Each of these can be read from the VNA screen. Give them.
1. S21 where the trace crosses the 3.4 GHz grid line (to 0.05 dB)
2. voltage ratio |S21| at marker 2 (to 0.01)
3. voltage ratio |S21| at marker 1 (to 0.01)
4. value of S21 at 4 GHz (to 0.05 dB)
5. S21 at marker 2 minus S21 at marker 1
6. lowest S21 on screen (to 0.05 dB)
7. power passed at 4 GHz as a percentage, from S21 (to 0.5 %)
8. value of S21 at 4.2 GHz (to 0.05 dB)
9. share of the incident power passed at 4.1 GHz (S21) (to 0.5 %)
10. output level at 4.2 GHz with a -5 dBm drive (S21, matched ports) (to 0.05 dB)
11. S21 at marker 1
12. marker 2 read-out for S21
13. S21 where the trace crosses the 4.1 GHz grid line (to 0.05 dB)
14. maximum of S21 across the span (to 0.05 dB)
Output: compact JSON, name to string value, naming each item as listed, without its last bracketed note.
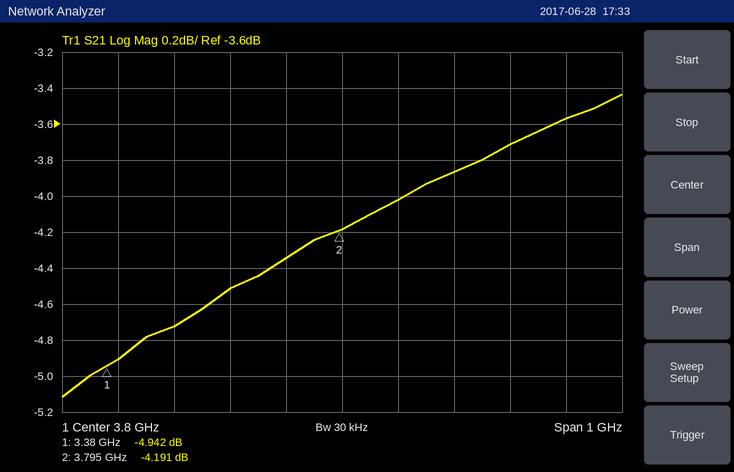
{"S21 where the trace crosses the 3.4 GHz grid line": "-4.90 dB", "voltage ratio |S21| at marker 2": "0.62", "voltage ratio |S21| at marker 1": "0.57", "value of S21 at 4 GHz": "-3.85 dB", "S21 at marker 2 minus S21 at marker 1": "0.751 dB", "lowest S21 on screen": "-5.10 dB", "power passed at 4 GHz as a percentage, from S21": "41.0 %", "value of S21 at 4.2 GHz": "-3.55 dB", "share of the incident power passed at 4.1 GHz (S21)": "42.5 %", "output level at 4.2 GHz with a -5 dBm drive (S21, matched ports)": "-8.55 dBm", "S21 at marker 1": "-4.942 dB", "marker 2 read-out for S21": "-4.191 dB", "S21 where the trace crosses the 4.1 GHz grid line": "-3.70 dB", "maximum of S21 across the span": "-3.45 dB"}
